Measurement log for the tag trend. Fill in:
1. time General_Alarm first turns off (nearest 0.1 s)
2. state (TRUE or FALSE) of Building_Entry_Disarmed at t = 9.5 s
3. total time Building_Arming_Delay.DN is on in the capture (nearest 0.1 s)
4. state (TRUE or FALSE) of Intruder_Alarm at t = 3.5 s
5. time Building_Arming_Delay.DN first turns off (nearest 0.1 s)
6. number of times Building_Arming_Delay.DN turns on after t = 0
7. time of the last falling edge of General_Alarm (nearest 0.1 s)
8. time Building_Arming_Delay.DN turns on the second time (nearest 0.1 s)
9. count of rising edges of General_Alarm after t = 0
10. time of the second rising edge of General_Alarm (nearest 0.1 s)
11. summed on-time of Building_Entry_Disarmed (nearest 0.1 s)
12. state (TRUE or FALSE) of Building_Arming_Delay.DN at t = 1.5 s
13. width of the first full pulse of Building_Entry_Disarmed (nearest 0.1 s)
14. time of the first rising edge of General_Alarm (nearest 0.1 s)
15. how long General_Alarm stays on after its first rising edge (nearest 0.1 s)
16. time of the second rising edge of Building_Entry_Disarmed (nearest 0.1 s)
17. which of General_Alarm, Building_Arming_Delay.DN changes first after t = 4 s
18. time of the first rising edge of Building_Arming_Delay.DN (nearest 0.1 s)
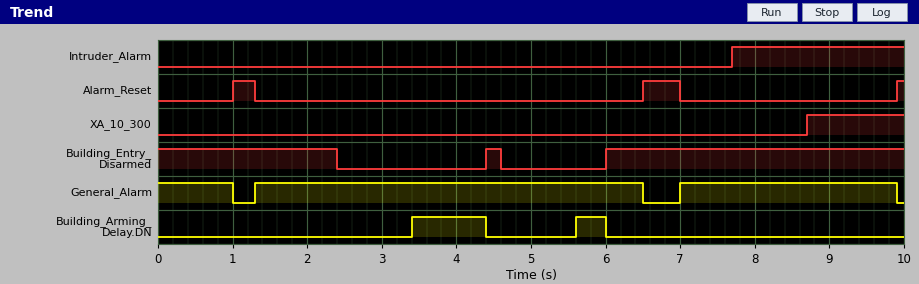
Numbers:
1.0 s
TRUE
1.4 s
FALSE
4.4 s
2
9.9 s
5.6 s
2
7.0 s
6.6 s
FALSE
0.2 s
1.3 s
5.2 s
6.0 s
Building_Arming_Delay.DN
3.4 s
